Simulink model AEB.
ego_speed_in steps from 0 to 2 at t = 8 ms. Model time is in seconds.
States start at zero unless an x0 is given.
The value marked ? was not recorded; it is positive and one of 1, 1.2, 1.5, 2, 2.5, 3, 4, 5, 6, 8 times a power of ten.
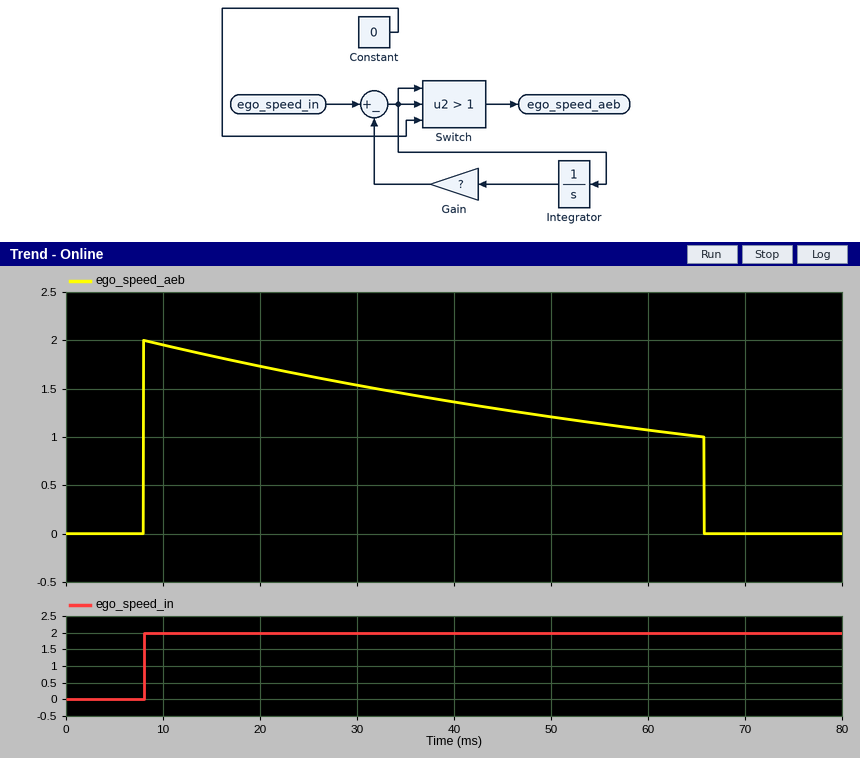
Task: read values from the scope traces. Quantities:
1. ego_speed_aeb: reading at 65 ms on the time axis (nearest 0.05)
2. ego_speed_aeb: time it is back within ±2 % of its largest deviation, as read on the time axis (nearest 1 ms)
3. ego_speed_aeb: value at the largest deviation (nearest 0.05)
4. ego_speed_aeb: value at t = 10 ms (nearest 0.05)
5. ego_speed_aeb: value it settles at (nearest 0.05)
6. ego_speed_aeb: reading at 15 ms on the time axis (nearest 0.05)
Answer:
1.00
66 ms
2.00
1.95
0.00
1.85
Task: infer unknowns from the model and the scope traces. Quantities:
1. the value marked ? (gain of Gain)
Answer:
12
